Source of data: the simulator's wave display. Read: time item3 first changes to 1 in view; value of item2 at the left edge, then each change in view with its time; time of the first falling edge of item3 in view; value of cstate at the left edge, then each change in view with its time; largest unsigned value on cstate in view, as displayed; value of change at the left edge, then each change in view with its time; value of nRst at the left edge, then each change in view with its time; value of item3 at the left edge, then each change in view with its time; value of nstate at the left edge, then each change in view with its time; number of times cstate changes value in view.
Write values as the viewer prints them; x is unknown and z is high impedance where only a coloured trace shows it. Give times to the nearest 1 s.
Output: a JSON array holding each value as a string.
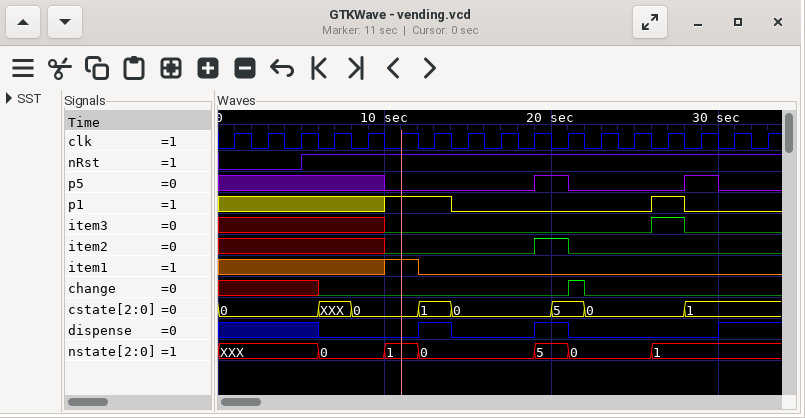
["26 s", "x, 0 at 10 s, 1 at 19 s, 0 at 21 s", "28 s", "0, XXX at 6 s, 0 at 8 s, 1 at 12 s, 0 at 14 s, 5 at 20 s, 0 at 22 s, 1 at 28 s", "5", "x, 0 at 6 s, 1 at 21 s, 0 at 22 s", "0, 1 at 5 s", "x, 0 at 10 s, 1 at 26 s, 0 at 28 s", "XXX, 0 at 6 s, 1 at 10 s, 0 at 12 s, 5 at 19 s, 0 at 21 s, 1 at 26 s", "7"]
